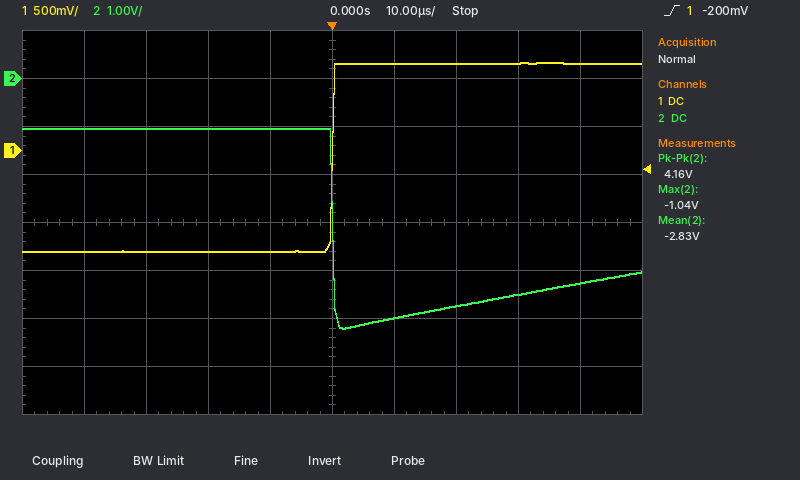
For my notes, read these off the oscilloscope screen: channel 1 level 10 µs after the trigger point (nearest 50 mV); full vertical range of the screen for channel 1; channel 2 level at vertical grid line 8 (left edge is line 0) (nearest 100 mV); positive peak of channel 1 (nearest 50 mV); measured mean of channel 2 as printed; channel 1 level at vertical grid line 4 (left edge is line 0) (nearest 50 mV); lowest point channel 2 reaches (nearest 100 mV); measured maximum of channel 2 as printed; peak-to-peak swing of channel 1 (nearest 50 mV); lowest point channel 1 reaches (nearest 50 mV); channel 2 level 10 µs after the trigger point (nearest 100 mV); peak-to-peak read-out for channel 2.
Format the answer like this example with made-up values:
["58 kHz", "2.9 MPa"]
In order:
["900 mV", "4 V", "-4.5 V", "900 mV", "-2.83 V", "-1.05 V", "-5.2 V", "-1.04 V", "1.95 V", "-1.05 V", "-5.0 V", "4.16 V"]
